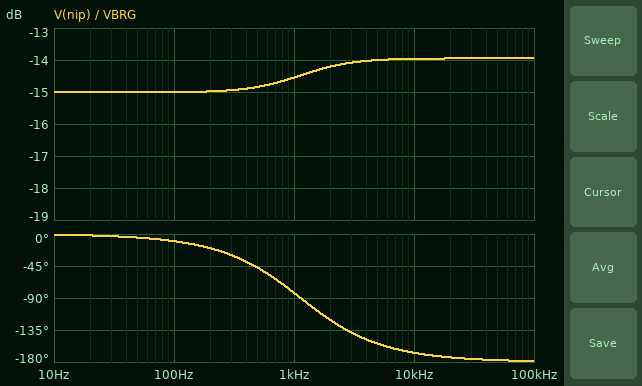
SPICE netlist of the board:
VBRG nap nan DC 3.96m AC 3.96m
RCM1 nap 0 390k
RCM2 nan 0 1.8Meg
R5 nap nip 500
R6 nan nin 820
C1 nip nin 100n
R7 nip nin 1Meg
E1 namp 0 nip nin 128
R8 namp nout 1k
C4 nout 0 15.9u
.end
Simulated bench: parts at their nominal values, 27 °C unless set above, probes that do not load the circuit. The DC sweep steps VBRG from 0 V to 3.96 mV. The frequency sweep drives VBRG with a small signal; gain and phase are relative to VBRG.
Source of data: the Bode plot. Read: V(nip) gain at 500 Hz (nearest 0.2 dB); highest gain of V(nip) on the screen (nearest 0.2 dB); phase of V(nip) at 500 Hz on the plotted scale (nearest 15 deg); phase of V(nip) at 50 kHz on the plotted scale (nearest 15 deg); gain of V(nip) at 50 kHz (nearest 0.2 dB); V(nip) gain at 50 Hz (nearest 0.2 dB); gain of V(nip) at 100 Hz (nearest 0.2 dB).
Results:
-14.8 dB
-14.0 dB
-45 deg
-180 deg
-14.0 dB
-15.0 dB
-15.0 dB
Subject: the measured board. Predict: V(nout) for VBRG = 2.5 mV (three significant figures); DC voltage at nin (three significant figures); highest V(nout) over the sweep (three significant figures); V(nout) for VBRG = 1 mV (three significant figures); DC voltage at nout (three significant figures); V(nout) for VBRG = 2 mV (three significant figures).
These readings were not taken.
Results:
320 mV
-3.25 mV
506 mV
128 mV
506 mV
256 mV
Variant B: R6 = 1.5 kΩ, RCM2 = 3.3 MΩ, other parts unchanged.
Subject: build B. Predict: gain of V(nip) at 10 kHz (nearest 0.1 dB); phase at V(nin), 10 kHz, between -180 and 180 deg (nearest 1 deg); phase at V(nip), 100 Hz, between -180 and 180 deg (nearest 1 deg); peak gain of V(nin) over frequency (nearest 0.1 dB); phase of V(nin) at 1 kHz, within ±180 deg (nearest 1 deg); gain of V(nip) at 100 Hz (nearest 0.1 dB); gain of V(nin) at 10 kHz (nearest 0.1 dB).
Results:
-16.8 dB
158 deg
-17 deg
-1.0 dB
140 deg
-19.5 dB
-15.9 dB
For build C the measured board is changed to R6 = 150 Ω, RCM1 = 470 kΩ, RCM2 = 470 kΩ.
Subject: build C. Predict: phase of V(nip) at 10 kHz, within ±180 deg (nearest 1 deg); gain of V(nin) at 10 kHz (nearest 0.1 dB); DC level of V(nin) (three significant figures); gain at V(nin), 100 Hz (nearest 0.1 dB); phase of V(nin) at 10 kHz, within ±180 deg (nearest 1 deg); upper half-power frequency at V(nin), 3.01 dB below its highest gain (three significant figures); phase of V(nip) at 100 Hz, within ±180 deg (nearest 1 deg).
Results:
-142 deg
-10.8 dB
-1.98 mV
-6.0 dB
169 deg
3.78 kHz
-4 deg
